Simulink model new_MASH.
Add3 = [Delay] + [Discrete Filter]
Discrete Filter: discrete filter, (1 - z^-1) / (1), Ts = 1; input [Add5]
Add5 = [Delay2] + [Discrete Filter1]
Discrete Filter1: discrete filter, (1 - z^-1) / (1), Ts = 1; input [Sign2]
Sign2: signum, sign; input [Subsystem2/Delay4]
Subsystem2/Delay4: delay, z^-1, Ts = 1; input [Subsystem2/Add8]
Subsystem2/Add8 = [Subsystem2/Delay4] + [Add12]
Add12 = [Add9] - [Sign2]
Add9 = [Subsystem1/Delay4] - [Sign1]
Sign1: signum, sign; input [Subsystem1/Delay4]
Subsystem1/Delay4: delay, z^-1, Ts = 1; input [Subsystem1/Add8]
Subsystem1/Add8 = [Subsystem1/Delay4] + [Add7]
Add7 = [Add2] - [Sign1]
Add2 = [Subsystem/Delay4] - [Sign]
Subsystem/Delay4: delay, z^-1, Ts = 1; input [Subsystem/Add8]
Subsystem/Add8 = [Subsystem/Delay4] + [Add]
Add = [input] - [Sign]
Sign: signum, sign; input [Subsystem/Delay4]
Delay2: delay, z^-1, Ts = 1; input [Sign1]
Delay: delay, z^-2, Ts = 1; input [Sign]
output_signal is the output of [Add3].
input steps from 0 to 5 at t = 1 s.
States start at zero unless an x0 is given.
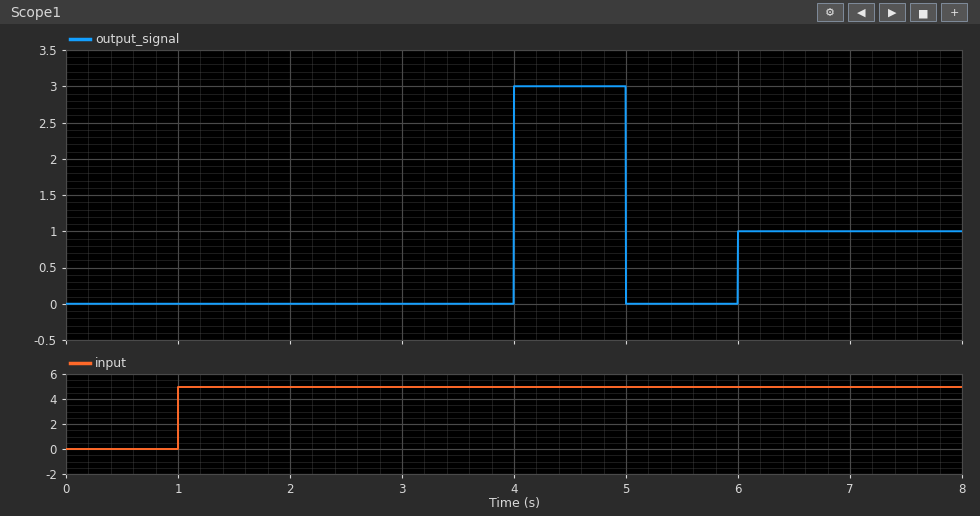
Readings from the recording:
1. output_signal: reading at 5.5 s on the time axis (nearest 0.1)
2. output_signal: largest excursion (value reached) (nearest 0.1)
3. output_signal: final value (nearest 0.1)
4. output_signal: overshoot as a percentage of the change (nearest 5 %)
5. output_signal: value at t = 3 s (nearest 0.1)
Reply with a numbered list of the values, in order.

1. 0.0
2. 3.0
3. 1.0
4. 200 %
5. 0.0
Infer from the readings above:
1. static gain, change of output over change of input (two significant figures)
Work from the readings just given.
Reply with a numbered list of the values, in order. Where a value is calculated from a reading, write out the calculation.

1. (1 - 0) / (5 - 0) = 0.20
